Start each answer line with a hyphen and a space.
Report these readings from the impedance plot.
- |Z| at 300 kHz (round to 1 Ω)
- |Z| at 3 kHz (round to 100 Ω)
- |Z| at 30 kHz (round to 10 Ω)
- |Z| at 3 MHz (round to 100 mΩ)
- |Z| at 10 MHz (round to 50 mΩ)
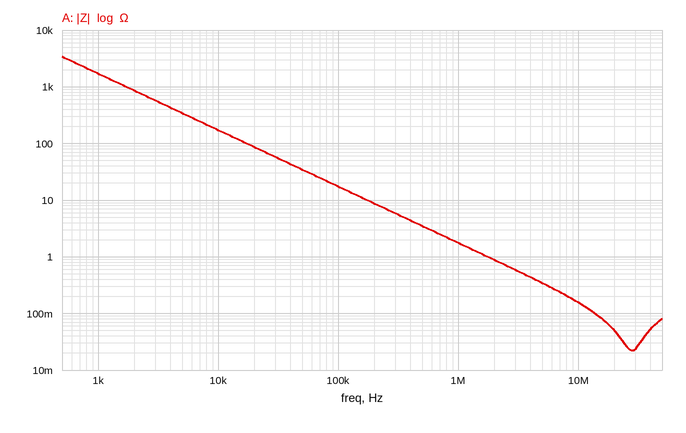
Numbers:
- 6 Ω
- 600 Ω
- 60 Ω
- 600 mΩ
- 150 mΩ
